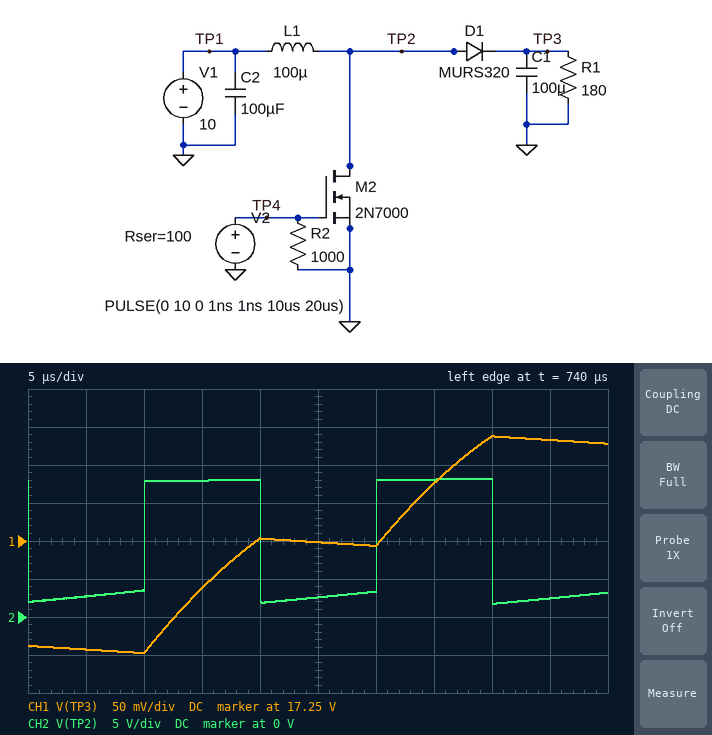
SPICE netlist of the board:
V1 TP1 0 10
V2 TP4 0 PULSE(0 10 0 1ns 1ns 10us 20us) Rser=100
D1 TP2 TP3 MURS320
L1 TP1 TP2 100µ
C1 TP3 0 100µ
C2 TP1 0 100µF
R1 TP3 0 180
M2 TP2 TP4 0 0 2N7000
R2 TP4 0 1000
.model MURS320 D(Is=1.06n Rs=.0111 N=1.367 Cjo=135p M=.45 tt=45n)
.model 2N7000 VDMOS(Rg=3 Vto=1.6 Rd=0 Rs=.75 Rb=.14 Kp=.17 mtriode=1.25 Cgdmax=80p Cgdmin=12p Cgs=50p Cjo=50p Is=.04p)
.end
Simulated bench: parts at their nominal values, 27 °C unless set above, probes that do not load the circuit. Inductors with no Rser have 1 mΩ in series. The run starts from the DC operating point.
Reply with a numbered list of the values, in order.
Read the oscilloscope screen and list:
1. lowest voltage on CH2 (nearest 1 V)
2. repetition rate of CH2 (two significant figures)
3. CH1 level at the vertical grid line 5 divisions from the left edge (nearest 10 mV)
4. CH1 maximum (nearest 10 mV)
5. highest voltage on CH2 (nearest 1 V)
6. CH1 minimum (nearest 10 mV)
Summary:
1. 2 V
2. 50 kHz
3. 17.25 V
4. 17.39 V
5. 18 V
6. 17.10 V
